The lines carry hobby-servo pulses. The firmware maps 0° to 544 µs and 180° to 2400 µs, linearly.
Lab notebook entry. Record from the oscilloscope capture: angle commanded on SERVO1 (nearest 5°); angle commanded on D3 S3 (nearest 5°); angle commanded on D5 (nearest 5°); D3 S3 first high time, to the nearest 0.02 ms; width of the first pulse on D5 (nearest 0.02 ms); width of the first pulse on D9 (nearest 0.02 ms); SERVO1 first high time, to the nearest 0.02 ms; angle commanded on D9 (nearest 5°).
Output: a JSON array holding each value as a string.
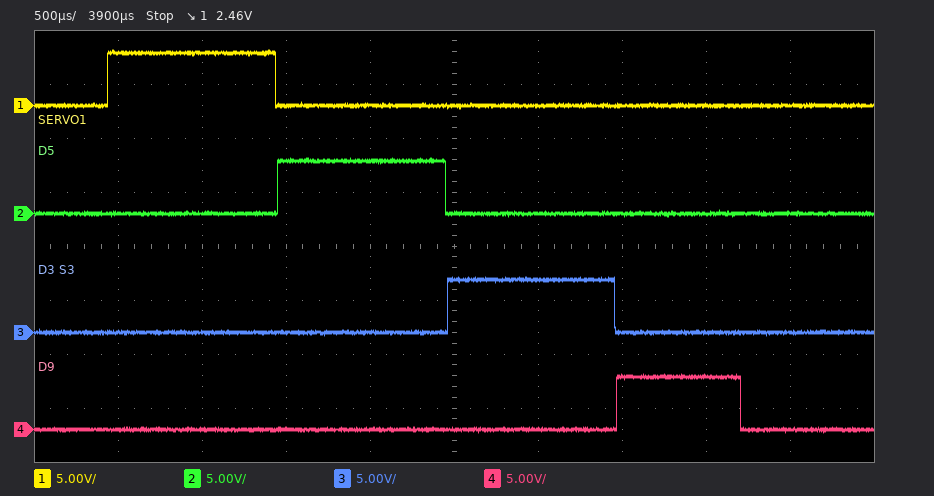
["45°", "45°", "45°", "1.00 ms", "1.00 ms", "0.74 ms", "1.00 ms", "20°"]
